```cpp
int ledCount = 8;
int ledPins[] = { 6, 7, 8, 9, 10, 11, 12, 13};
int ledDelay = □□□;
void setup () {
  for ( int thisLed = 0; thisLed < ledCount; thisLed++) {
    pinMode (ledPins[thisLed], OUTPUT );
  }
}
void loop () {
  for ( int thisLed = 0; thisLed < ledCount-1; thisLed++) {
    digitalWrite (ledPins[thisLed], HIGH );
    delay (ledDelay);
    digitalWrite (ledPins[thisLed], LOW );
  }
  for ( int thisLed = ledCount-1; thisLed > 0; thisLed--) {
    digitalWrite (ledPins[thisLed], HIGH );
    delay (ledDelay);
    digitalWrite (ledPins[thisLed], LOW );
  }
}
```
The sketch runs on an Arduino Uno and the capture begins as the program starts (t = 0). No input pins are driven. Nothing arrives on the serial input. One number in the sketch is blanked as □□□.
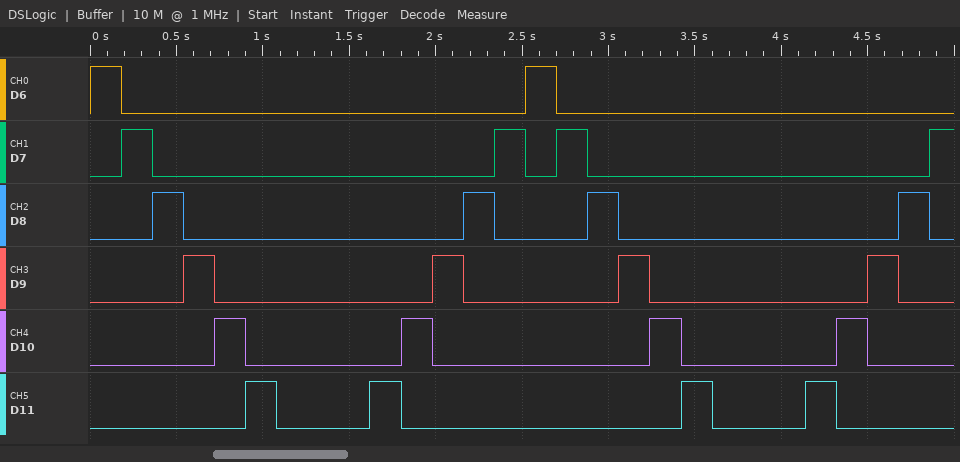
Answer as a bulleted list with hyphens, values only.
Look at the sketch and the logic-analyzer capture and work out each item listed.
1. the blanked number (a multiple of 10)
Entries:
- 180
